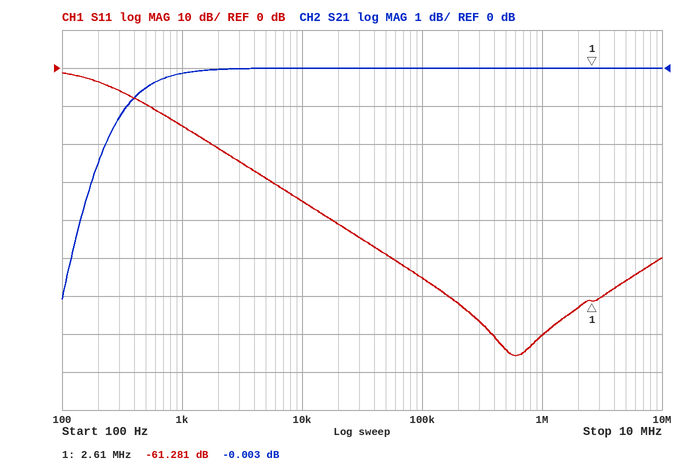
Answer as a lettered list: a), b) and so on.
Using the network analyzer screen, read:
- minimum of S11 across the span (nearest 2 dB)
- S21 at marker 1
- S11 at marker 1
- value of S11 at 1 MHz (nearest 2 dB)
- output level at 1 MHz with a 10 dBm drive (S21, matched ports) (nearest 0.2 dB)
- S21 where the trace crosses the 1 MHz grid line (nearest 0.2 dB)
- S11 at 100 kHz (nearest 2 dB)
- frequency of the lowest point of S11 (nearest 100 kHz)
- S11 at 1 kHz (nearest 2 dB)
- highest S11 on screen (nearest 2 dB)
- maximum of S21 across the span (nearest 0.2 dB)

a) -76 dB
b) -0.003 dB
c) -61.281 dB
d) -70 dB
e) 10.0 dBm
f) 0.0 dB
g) -56 dB
h) 600 kHz
i) -16 dB
j) -2 dB
k) 0.0 dB
